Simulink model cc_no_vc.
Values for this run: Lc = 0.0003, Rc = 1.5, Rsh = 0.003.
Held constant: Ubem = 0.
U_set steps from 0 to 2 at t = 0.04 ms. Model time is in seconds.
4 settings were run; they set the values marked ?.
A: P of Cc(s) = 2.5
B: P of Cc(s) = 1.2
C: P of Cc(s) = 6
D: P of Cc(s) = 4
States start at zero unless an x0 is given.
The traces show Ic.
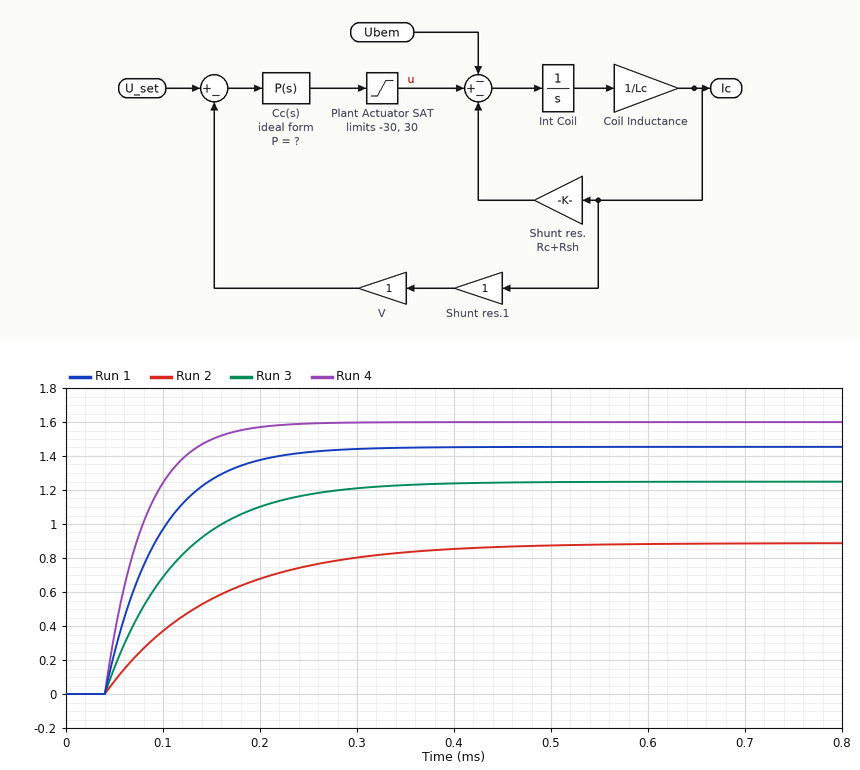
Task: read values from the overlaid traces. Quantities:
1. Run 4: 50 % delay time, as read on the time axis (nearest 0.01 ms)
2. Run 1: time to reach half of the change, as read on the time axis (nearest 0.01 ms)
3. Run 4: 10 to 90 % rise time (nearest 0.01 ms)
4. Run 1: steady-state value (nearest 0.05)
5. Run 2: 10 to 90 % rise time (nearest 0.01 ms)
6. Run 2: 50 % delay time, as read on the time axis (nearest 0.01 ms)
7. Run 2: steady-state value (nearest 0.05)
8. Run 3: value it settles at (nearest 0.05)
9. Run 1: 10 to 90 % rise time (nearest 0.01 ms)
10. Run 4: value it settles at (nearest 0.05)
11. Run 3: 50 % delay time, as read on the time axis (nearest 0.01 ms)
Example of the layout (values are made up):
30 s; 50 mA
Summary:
0.07 ms; 0.08 ms; 0.09 ms; 1.45; 0.24 ms; 0.12 ms; 0.90; 1.25; 0.12 ms; 1.60; 0.09 ms
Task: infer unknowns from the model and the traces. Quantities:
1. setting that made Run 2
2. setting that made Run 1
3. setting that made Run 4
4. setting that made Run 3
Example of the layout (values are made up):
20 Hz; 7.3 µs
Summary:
B; D; C; A
